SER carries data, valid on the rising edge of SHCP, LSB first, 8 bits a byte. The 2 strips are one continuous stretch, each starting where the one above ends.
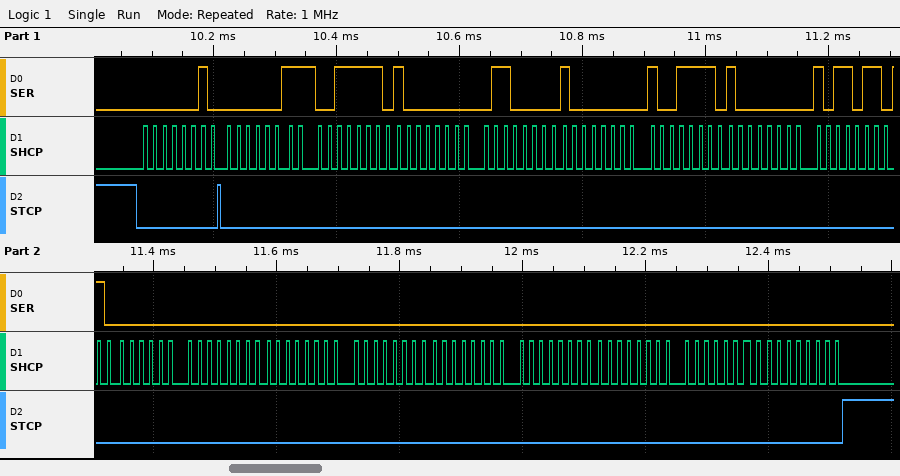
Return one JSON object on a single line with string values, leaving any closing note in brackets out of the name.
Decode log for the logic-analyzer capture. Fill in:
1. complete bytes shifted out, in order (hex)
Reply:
{"complete bytes shifted out, in order": "0x40 0xC0 0x7C 0x01 0x06 0x01 0x79 0x01 0x6D 0x01 0x00 0x00 0x00 0x00 0x00 0x00 0x00 0x00"}
